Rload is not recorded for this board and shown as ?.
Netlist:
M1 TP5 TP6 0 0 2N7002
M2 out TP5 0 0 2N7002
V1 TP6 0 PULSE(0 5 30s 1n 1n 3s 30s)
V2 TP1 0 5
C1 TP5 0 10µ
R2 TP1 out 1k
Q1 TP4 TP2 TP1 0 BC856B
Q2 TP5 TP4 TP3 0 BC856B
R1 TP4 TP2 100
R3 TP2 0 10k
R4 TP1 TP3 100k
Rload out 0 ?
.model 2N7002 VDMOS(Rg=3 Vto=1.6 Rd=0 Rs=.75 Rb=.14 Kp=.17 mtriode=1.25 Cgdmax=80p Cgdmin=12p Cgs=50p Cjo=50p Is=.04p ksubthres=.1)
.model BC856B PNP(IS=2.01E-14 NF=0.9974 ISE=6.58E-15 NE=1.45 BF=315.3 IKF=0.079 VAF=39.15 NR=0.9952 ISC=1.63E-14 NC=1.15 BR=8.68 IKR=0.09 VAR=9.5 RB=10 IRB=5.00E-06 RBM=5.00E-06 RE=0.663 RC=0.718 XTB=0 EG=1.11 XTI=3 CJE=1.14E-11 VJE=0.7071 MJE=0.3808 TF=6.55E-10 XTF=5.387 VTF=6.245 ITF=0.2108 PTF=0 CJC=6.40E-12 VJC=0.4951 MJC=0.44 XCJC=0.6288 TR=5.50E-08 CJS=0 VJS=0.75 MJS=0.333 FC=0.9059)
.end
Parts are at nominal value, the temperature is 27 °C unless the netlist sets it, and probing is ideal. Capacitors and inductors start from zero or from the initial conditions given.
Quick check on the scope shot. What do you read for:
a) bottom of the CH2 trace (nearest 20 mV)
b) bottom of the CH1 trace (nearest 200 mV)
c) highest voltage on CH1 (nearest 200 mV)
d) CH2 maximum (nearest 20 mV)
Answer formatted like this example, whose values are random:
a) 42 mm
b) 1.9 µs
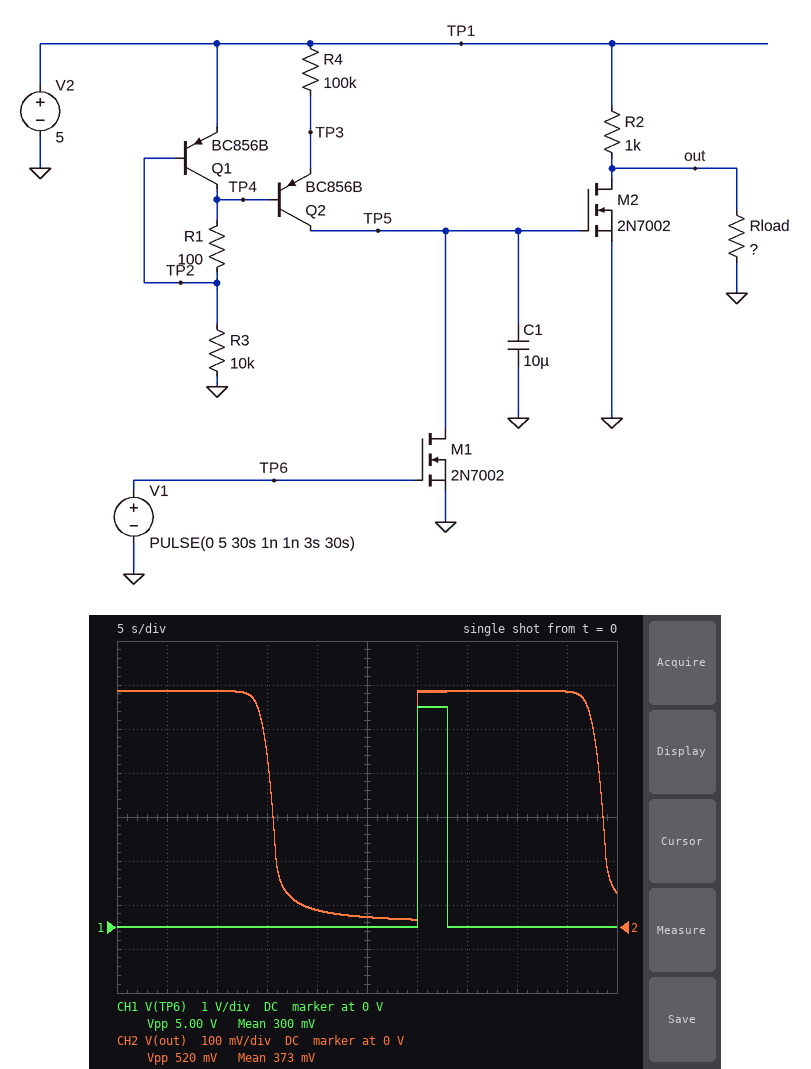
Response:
a) 20 mV
b) 0 V
c) 5.0 V
d) 540 mV
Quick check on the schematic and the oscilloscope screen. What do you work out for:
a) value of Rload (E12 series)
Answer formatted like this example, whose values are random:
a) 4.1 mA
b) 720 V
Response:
a) 120 Ω
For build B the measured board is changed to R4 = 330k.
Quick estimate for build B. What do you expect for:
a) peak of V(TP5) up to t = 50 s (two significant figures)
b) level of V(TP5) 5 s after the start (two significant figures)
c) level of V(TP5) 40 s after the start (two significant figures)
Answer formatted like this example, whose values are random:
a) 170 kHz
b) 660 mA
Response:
a) 1.3 V
b) 210 mV
c) 290 mV
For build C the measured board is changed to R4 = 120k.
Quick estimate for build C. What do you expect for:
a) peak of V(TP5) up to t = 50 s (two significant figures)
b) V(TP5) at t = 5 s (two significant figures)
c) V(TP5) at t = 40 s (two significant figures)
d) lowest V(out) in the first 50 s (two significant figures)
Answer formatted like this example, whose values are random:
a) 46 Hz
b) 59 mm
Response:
a) 2.9 V
b) 490 mV
c) 680 mV
d) 21 mV
